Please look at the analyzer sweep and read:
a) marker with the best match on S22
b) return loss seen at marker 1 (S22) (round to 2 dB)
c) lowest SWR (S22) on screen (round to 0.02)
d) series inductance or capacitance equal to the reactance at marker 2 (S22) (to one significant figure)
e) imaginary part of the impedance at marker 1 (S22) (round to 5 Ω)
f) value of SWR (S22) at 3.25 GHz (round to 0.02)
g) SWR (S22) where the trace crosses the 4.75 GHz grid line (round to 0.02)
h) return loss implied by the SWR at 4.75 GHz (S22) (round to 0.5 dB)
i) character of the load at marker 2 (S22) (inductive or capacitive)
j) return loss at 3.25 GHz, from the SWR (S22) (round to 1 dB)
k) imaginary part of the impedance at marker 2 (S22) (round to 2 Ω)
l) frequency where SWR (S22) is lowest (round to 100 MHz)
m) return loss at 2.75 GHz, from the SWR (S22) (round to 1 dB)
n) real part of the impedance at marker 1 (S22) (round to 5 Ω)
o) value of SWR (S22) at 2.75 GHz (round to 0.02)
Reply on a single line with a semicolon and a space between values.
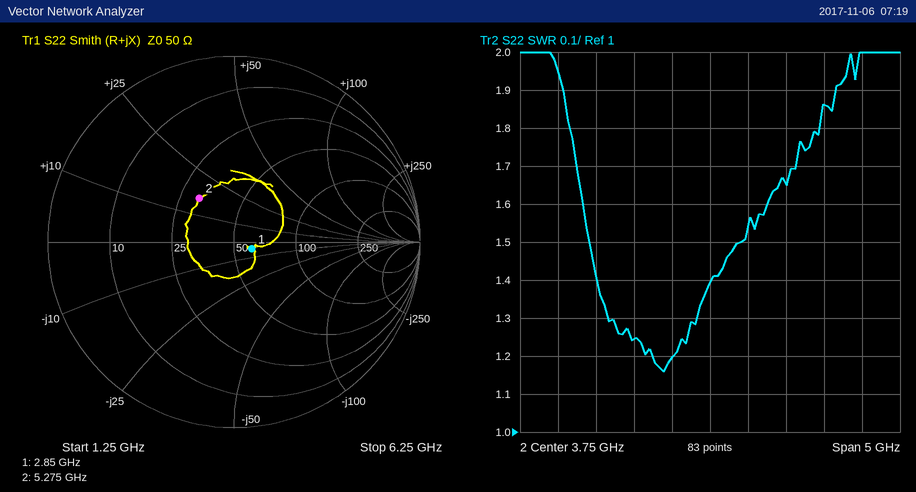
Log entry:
marker 1; 20 dB; 1.16; 500 pH; -5 Ω; 1.20; 1.66; 12.0 dB; inductive; 21 dB; +16 Ω; 3.1 GHz; 19 dB; 60 Ω; 1.24
